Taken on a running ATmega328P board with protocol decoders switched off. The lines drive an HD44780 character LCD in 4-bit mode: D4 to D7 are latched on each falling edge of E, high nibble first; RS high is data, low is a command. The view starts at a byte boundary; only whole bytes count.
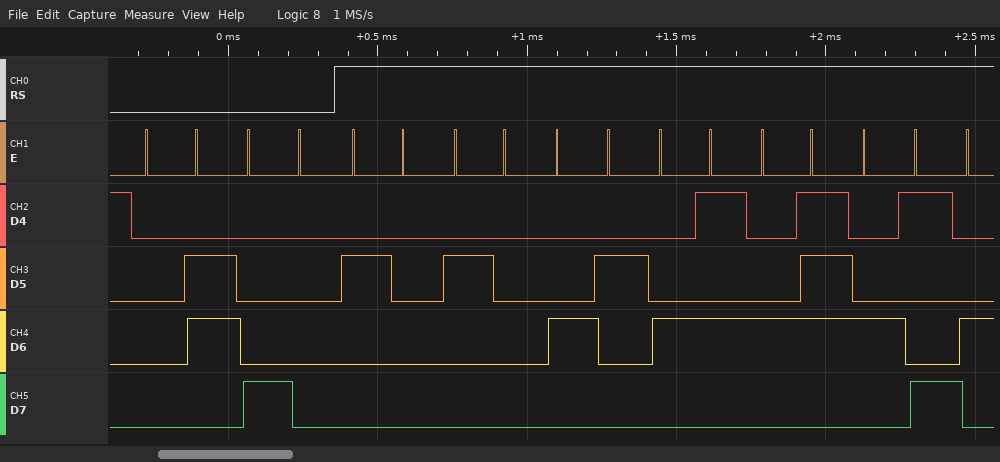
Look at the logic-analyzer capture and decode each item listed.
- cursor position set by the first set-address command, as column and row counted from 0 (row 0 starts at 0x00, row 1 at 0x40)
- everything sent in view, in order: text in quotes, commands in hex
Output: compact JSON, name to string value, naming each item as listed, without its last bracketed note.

{"cursor position set by the first set-address command, as column and row counted from 0": "column 0, row 0", "everything sent in view, in order: text in quotes, commands in hex": "0x06 0x80 \"  BEGI\""}
